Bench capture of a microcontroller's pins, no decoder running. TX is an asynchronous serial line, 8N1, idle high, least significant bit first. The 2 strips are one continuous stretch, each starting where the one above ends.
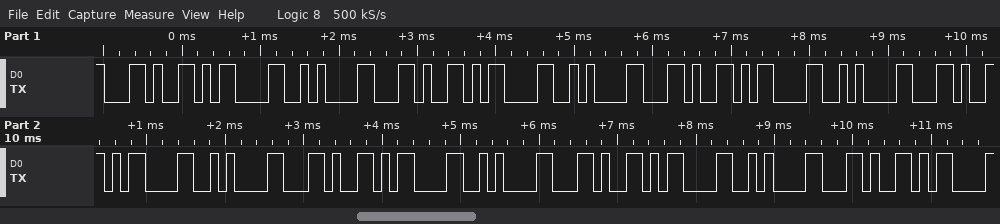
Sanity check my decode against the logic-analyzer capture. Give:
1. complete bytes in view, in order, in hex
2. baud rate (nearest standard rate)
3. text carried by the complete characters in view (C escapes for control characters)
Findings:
2C 0D 0A 2C 0D 0A 2C 0D 0A 2C 0D 0A 2C 0D 0A 2C 0D 0A 2C 0D
9600 baud
",\r\n,\r\n,\r\n,\r\n,\r\n,\r\n,\r"
